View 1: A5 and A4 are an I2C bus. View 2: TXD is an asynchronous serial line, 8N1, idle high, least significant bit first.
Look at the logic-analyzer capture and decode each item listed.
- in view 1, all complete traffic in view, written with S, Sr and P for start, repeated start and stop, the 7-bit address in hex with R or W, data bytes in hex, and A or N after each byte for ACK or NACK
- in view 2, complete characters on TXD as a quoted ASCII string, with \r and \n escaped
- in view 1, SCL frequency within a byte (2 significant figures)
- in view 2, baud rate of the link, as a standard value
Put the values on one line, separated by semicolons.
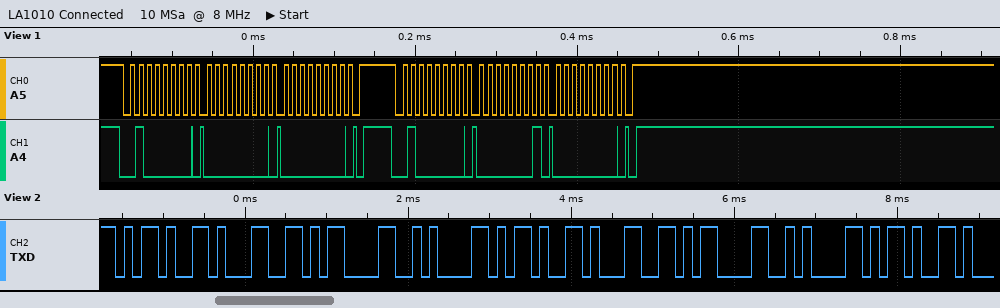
S 20W A 00 A 00 A P S 20W A 01 A 00 A P; "-1\r\n-1\r\n-"; 100 kHz; 9600 baud
